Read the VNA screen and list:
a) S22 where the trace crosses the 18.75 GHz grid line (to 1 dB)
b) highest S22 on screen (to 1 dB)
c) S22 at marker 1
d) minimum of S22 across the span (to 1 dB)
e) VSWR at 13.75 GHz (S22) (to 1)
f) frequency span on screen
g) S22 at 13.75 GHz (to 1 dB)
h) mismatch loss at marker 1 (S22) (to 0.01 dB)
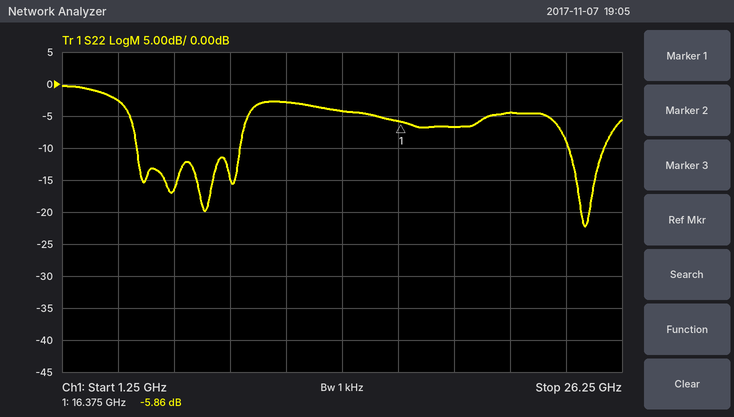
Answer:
-7 dB
0 dB
-5.86 dB
-22 dB
4
25 GHz
-4 dB
1.30 dB
